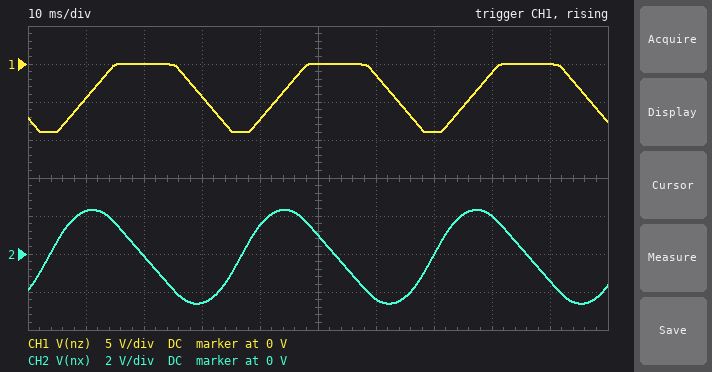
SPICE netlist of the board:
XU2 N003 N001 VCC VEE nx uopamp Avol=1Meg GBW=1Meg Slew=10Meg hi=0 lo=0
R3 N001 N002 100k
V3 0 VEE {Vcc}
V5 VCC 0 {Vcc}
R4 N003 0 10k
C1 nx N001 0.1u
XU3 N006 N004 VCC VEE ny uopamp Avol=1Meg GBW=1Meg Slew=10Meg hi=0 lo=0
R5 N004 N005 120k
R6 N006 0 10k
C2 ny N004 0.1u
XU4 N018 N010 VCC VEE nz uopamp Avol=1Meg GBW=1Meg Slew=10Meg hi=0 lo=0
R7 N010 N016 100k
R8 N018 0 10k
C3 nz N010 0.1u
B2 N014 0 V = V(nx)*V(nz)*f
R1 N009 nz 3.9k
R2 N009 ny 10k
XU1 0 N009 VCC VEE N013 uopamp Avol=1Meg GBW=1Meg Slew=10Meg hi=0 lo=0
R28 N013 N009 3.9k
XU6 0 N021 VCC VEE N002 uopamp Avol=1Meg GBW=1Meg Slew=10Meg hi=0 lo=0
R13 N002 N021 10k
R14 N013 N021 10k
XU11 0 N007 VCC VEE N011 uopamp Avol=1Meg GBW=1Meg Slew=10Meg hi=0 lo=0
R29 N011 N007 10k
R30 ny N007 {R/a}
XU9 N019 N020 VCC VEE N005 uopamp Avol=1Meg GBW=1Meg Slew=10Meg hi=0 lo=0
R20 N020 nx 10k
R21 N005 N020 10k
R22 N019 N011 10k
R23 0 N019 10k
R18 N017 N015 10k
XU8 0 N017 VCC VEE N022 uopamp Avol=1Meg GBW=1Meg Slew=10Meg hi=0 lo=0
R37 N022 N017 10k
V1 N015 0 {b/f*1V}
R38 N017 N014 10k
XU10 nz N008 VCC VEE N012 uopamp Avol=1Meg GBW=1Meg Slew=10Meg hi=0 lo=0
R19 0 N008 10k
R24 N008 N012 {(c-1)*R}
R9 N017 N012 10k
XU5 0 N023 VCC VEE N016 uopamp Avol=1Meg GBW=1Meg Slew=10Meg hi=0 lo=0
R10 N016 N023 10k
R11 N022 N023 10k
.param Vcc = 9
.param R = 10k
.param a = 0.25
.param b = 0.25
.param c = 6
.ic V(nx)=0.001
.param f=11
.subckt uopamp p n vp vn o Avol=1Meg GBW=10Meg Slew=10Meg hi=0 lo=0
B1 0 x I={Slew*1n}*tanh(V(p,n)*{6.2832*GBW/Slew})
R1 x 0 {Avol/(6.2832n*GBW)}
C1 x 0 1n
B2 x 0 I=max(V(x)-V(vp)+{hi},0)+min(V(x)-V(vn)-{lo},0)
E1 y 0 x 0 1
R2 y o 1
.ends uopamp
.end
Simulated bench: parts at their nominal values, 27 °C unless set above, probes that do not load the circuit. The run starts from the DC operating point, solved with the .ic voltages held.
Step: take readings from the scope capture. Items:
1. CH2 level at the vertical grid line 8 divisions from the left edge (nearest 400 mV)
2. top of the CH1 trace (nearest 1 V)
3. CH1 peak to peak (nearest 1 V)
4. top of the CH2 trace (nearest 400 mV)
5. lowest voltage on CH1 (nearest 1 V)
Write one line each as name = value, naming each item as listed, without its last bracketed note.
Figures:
CH2 level at the vertical grid line 8 divisions from the left edge = 2.0 V
top of the CH1 trace = 0 V
CH1 peak to peak = 9 V
top of the CH2 trace = 2.4 V
lowest voltage on CH1 = -9 V
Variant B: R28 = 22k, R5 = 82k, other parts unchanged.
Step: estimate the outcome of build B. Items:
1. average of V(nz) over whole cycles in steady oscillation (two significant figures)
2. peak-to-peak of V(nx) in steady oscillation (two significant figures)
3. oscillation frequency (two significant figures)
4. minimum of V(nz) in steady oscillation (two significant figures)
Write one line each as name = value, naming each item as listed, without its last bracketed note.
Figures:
average of V(nz) over whole cycles in steady oscillation = -30 mV
peak-to-peak of V(nx) in steady oscillation = 1.7 V
oscillation frequency = 14 Hz
minimum of V(nz) in steady oscillation = -220 mV
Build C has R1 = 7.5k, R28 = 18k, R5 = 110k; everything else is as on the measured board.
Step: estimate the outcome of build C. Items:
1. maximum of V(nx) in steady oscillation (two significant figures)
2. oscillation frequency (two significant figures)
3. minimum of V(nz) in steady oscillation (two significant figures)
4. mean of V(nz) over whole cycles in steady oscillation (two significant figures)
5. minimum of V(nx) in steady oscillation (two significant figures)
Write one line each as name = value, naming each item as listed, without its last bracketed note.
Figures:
maximum of V(nx) in steady oscillation = 780 mV
oscillation frequency = 11 Hz
minimum of V(nz) in steady oscillation = -540 mV
mean of V(nz) over whole cycles in steady oscillation = -46 mV
minimum of V(nx) in steady oscillation = -960 mV
